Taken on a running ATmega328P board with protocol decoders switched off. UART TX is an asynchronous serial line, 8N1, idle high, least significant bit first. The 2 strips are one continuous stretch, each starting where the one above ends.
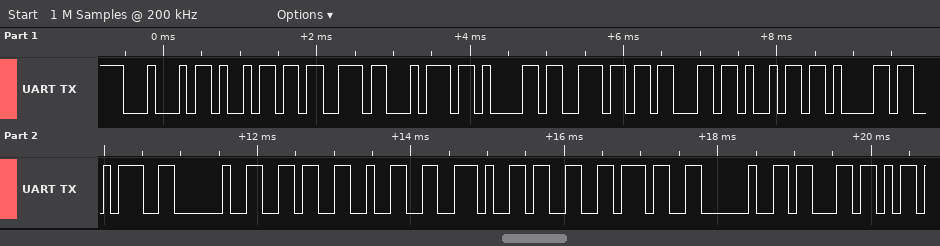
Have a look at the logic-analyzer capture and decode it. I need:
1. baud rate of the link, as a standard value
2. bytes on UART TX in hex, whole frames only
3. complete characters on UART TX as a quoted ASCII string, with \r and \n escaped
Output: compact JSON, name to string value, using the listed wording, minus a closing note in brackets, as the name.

{"baud rate of the link, as a standard value": "9600 baud", "bytes on UART TX in hex, whole frames only": "44 69 73 74 61 6E 63 69 61 3A 20 36 32 2E 33 37 20 63", "complete characters on UART TX as a quoted ASCII string, with \\r and \\n escaped": "\"Distancia: 62.37 c\""}
